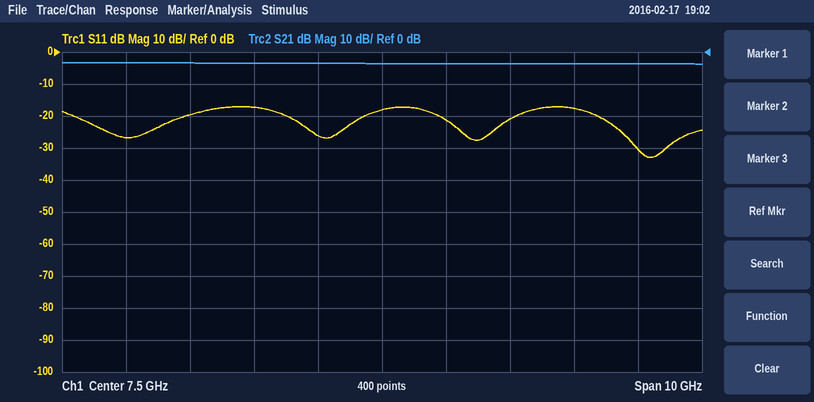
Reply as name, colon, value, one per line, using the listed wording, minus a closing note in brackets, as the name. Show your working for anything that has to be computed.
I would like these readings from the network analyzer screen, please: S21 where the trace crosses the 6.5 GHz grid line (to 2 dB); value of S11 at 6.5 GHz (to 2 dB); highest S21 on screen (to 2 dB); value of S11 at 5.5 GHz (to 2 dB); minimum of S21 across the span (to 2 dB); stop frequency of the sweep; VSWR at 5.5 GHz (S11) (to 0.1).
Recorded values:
S21 where the trace crosses the 6.5 GHz grid line: -4 dB
value of S11 at 6.5 GHz: -26 dB
highest S21 on screen: -4 dB
value of S11 at 5.5 GHz: -18 dB
minimum of S21 across the span: -4 dB
stop frequency of the sweep: 12.5 GHz
VSWR at 5.5 GHz (S11): |Γ| = 10^(-18/20) = 0.1259; VSWR = (1 + 0.1259)/(1 − 0.1259) ≈ 1.3
